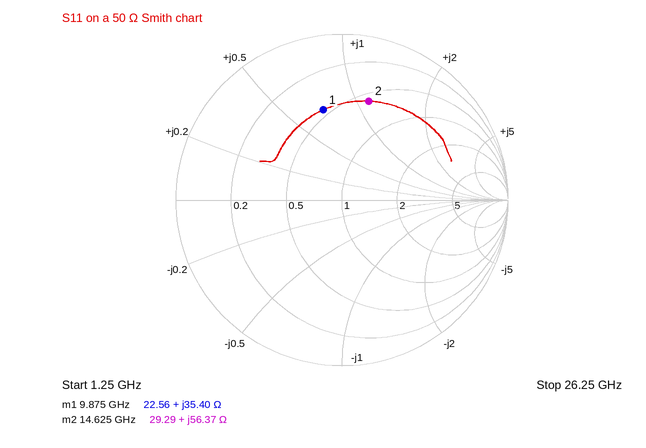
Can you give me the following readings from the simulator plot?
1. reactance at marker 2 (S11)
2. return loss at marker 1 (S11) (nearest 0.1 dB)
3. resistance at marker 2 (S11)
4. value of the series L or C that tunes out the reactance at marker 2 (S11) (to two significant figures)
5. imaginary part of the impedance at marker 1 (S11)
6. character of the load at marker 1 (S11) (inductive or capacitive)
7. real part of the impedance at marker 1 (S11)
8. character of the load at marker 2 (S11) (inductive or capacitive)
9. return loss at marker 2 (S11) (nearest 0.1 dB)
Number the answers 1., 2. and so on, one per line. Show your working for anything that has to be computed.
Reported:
1. +56.37 Ω
2. 5.1 dB
3. 29.29 Ω
4. C = 1/(2π × 14.625 GHz × 56.37 Ω) ≈ 193 fF, so 190 fF to two significant figures
5. +35.40 Ω
6. inductive
7. 22.56 Ω
8. inductive
9. 4.2 dB
